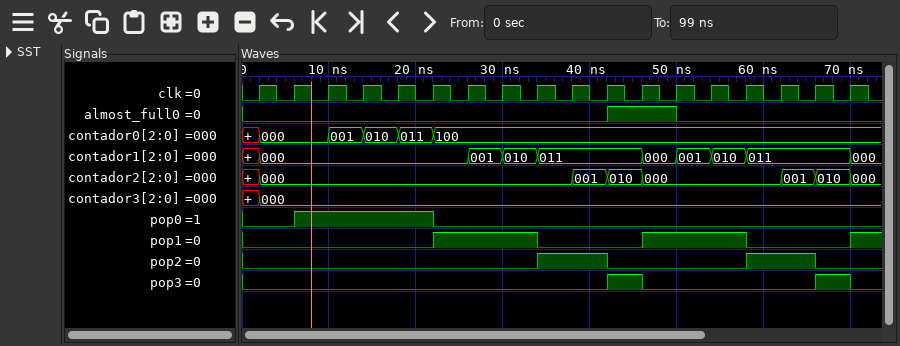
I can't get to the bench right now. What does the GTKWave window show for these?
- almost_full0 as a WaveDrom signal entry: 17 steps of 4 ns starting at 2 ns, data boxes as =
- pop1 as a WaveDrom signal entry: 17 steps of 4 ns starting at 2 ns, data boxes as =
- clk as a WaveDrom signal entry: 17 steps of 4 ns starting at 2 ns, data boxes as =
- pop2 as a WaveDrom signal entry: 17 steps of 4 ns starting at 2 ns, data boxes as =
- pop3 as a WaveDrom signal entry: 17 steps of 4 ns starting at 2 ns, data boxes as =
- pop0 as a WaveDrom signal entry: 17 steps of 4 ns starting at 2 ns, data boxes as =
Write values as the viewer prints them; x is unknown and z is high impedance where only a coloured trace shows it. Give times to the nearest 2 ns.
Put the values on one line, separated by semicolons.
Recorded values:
{name: 'almost_full0', wave: '0.........1.0....'}; {name: 'pop1', wave: '0....1..0..1..0..'}; {name: 'clk', wave: 'p................'}; {name: 'pop2', wave: '0.......1.0...1.0'}; {name: 'pop3', wave: '0.........10....1'}; {name: 'pop0', wave: '01...0...........'}
